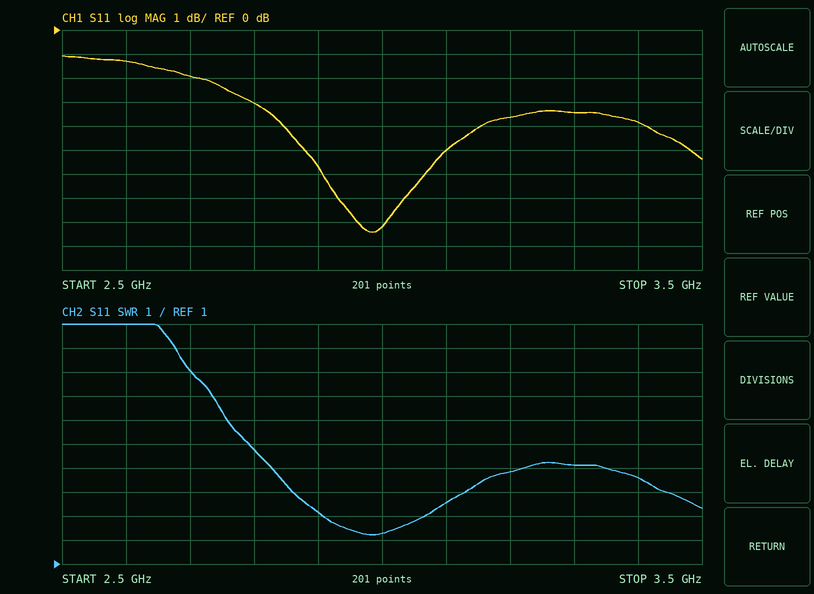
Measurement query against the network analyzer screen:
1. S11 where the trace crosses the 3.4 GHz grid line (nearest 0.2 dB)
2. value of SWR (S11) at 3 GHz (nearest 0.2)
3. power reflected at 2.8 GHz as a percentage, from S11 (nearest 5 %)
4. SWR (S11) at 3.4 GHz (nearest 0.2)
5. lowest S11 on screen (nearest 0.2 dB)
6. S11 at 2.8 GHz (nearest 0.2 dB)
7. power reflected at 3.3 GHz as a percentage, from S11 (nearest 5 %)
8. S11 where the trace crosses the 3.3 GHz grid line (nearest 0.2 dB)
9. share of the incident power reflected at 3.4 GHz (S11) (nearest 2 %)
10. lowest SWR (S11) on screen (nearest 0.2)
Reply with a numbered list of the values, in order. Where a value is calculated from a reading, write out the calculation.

1. -3.8 dB
2. 2.2
3. 10^(-3/10) ≈ 50 %
4. 4.6
5. -8.4 dB
6. -3.0 dB
7. 10^(-3.4/10) ≈ 45.7 %, so 45 % to the nearest 5 %
8. -3.4 dB
9. 10^(-3.8/10) ≈ 42 %
10. 2.2
